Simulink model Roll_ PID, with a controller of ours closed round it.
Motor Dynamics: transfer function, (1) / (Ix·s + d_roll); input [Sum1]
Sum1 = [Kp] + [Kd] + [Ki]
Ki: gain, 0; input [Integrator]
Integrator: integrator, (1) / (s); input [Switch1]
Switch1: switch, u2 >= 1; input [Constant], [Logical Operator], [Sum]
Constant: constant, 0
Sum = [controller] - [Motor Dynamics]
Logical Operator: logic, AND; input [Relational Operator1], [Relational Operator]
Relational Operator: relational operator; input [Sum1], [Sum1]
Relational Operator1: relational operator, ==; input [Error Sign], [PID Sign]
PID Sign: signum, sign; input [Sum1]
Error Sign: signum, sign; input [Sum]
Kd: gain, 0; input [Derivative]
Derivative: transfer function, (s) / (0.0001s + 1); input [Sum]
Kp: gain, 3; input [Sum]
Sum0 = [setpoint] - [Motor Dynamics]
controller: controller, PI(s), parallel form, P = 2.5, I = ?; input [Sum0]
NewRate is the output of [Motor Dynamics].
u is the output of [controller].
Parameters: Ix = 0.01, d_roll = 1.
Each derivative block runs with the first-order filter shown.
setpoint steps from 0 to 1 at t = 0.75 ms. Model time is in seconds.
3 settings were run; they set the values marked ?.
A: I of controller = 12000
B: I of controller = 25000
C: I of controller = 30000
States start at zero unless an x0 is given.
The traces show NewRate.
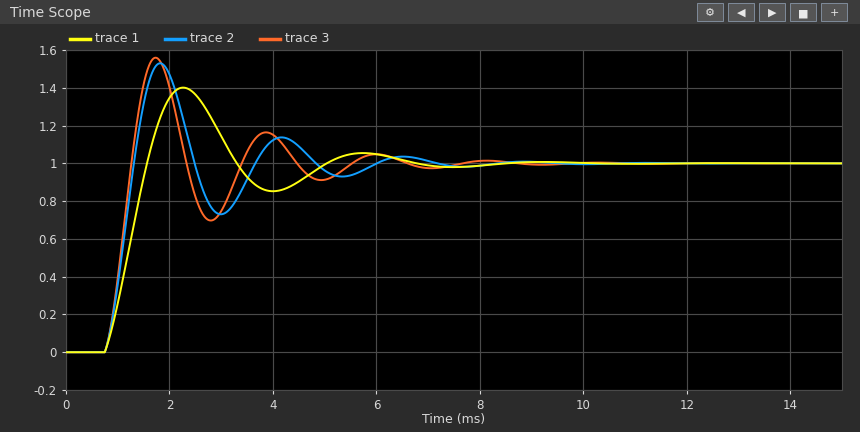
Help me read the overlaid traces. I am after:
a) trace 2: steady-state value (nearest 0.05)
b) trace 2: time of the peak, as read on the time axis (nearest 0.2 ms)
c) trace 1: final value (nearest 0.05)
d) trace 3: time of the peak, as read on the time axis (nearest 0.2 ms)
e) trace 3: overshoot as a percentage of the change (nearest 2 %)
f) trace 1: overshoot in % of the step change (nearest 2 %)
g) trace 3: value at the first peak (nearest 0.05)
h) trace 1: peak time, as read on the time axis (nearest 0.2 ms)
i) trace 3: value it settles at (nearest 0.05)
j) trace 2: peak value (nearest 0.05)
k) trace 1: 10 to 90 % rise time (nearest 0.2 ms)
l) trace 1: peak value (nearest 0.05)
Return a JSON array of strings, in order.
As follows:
["1.00", "1.8 ms", "1.00", "1.8 ms", "56 %", "40 %", "1.55", "2.2 ms", "1.00", "1.55", "0.6 ms", "1.40"]
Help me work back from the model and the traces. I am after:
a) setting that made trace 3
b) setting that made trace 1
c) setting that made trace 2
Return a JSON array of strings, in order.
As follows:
["C", "A", "B"]
